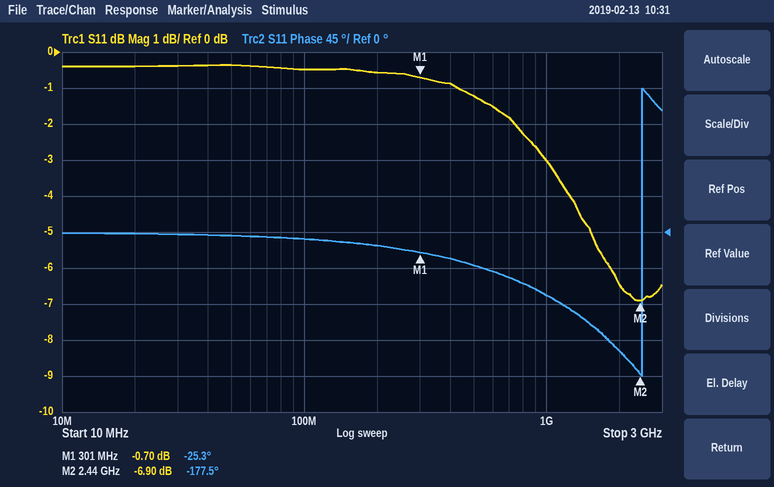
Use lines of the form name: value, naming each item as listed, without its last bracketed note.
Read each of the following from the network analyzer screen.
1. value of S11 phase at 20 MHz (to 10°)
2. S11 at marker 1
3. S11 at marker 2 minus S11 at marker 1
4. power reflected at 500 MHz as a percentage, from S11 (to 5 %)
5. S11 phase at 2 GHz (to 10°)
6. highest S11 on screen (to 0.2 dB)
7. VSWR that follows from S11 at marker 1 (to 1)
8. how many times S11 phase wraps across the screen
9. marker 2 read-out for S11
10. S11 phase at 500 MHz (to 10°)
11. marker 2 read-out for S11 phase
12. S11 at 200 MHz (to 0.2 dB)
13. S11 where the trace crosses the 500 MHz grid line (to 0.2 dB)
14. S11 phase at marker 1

value of S11 phase at 20 MHz: 0°
S11 at marker 1: -0.70 dB
S11 at marker 2 minus S11 at marker 1: -6.20 dB
power reflected at 500 MHz as a percentage, from S11: 75 %
S11 phase at 2 GHz: -150°
highest S11 on screen: -0.4 dB
VSWR that follows from S11 at marker 1: 25
how many times S11 phase wraps across the screen: 1
marker 2 read-out for S11: -6.90 dB
S11 phase at 500 MHz: -40°
marker 2 read-out for S11 phase: -177.5°
S11 at 200 MHz: -0.6 dB
S11 where the trace crosses the 500 MHz grid line: -1.2 dB
S11 phase at marker 1: -25.3°
